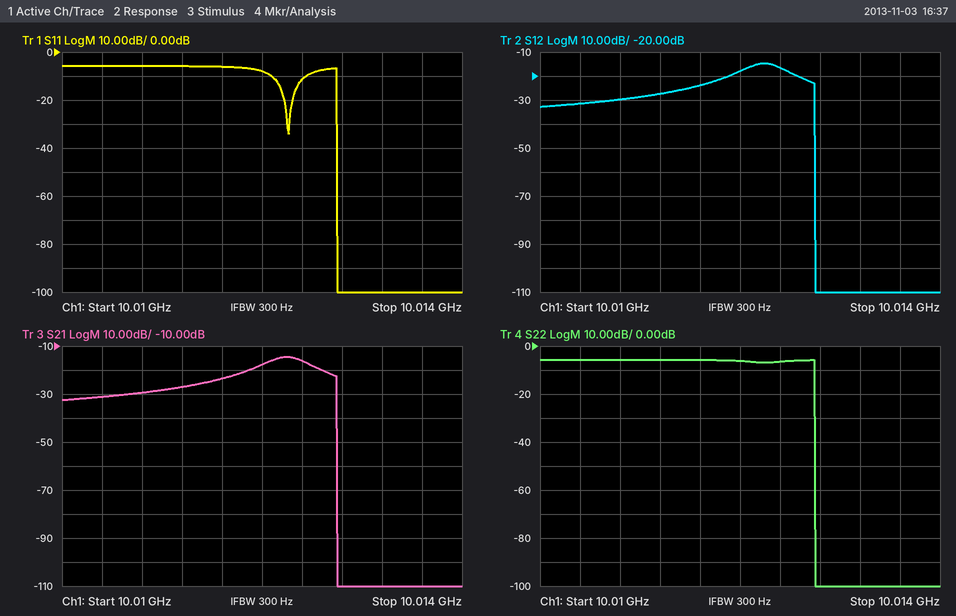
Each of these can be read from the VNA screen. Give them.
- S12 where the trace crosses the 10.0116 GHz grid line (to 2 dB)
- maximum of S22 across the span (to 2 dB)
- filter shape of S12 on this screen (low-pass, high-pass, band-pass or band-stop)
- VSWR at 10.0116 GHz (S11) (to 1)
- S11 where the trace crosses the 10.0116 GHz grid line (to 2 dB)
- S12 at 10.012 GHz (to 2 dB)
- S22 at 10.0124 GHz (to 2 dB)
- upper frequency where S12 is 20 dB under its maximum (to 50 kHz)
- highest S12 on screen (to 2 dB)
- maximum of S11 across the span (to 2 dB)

-24 dB
-6 dB
band-pass
3
-6 dB
-18 dB
-6 dB
10.01275 GHz
-14 dB
-6 dB
